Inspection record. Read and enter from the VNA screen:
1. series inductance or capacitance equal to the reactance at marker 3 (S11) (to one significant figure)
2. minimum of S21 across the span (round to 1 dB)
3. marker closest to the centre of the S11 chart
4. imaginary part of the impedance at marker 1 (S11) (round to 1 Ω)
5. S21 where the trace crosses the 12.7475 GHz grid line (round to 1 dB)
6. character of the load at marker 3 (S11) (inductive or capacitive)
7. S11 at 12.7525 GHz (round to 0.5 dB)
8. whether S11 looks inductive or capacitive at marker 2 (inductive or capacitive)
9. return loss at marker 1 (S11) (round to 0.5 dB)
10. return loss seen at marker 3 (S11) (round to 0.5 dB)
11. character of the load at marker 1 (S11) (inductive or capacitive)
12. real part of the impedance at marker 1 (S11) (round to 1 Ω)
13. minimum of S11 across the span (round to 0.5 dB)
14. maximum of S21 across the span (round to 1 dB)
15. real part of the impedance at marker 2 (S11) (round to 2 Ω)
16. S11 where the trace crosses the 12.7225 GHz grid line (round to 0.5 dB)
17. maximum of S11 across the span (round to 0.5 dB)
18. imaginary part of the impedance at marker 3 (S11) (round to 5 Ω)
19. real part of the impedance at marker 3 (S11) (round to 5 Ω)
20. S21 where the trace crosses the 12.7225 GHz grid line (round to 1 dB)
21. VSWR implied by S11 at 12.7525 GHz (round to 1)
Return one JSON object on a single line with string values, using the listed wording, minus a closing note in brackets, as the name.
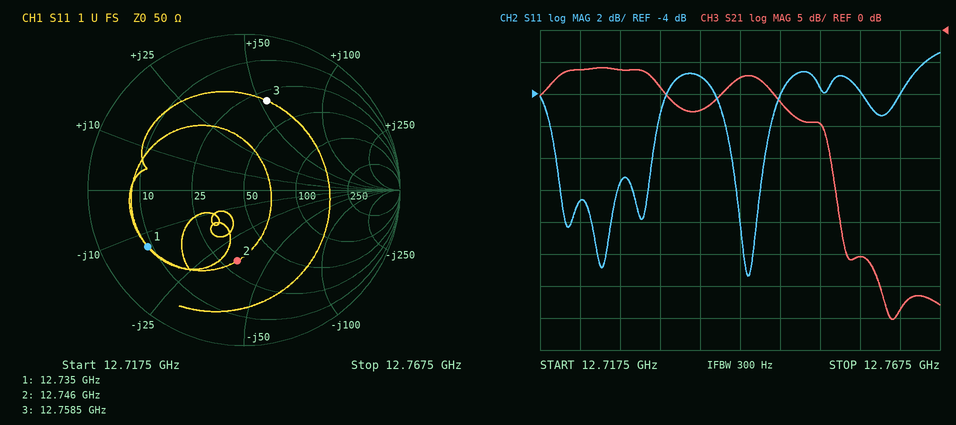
{"series inductance or capacitance equal to the reactance at marker 3 (S11)": "700 pH", "minimum of S21 across the span": "-45 dB", "marker closest to the centre of the S11 chart": "marker 2", "imaginary part of the impedance at marker 1 (S11)": "-13 Ω", "S21 where the trace crosses the 12.7475 GHz grid line": "-11 dB", "character of the load at marker 3 (S11)": "inductive", "S11 at 12.7525 GHz": "-3.5 dB", "whether S11 looks inductive or capacitive at marker 2": "capacitive", "return loss at marker 1 (S11)": "3.0 dB", "return loss seen at marker 3 (S11)": "4.5 dB", "character of the load at marker 1 (S11)": "capacitive", "real part of the impedance at marker 1 (S11)": "9 Ω", "minimum of S11 across the span": "-15.5 dB", "maximum of S21 across the span": "-6 dB", "real part of the impedance at marker 2 (S11)": "30 Ω", "S11 where the trace crosses the 12.7225 GHz grid line": "-10.5 dB", "maximum of S11 across the span": "-1.5 dB", "imaginary part of the impedance at marker 3 (S11)": "+55 Ω", "real part of the impedance at marker 3 (S11)": "30 Ω", "S21 where the trace crosses the 12.7225 GHz grid line": "-6 dB", "VSWR implied by S11 at 12.7525 GHz": "5"}
